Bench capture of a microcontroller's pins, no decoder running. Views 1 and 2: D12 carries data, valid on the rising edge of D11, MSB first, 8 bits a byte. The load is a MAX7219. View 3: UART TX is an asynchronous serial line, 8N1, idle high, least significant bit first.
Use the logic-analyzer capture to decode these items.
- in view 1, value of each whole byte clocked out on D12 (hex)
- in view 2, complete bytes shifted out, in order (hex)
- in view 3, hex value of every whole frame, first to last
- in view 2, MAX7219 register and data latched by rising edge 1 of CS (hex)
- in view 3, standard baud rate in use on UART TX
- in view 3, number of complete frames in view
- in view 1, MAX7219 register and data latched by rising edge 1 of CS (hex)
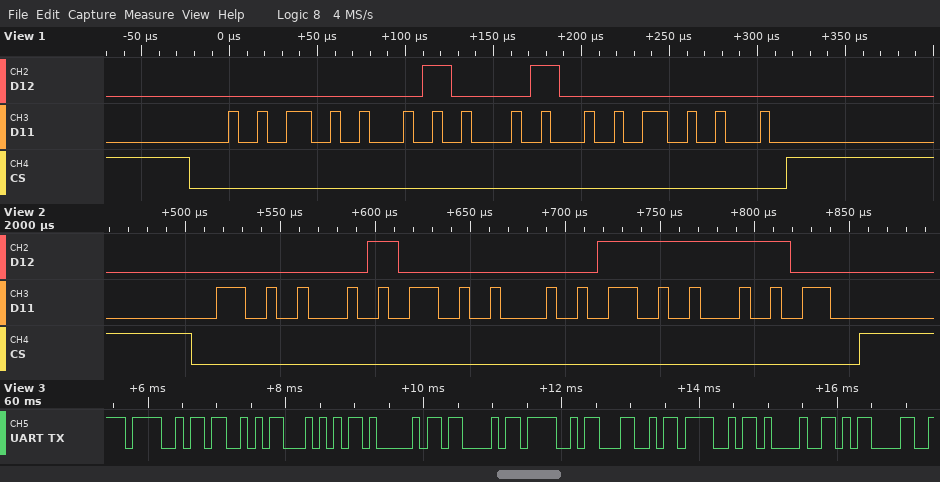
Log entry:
02 40
08 3E
4F 53 54 41 43 4F 4C 4F 21 0D
register 0x8, data 0x3E
9600 baud
10
register 0x2, data 0x40
